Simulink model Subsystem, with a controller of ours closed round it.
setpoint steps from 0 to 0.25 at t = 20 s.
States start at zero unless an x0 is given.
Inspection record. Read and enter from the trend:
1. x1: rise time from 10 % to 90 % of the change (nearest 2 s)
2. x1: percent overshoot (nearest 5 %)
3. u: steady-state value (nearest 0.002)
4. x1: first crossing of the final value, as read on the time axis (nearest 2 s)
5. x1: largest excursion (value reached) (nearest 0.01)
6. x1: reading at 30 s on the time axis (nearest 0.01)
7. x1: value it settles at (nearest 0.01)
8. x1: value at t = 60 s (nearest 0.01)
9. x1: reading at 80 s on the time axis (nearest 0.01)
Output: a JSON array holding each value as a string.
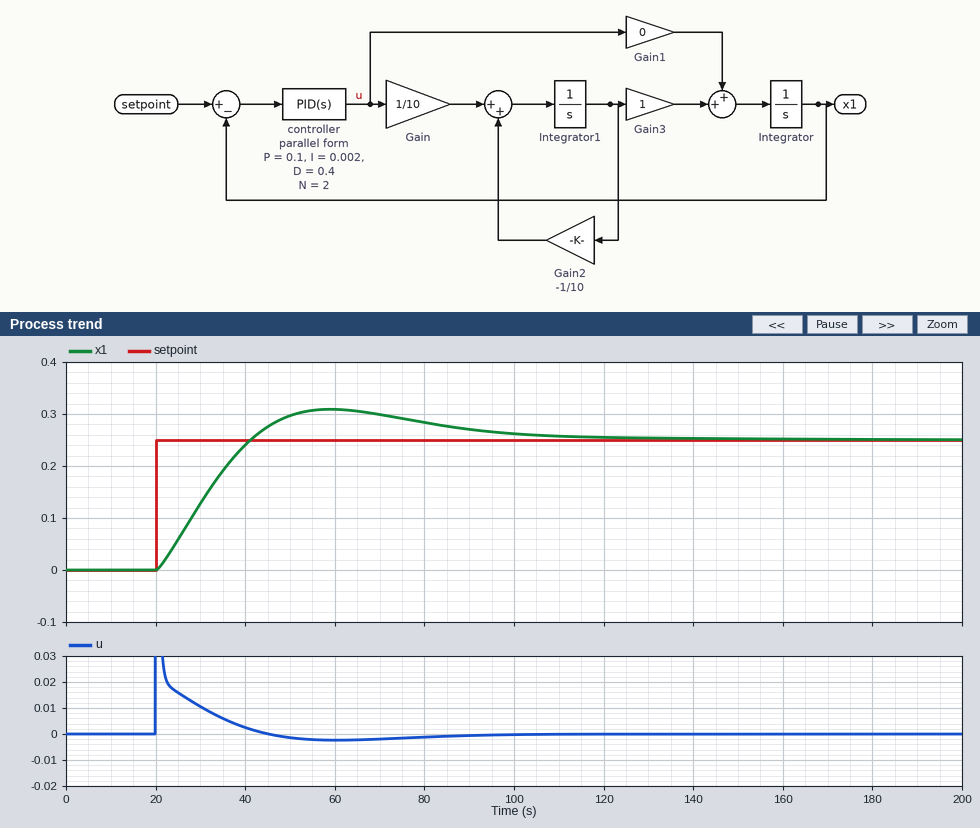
["16 s", "25 %", "0.000", "42 s", "0.31", "0.13", "0.25", "0.31", "0.28"]
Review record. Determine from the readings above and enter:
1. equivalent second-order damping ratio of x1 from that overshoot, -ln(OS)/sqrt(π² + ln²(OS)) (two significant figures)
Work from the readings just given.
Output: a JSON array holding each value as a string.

["0.40"]
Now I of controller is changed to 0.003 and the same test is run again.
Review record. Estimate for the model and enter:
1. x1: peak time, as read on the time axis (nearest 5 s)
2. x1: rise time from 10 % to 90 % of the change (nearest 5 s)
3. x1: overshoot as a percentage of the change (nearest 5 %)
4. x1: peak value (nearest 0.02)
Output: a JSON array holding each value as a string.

["60 s", "15 s", "30 %", "0.32"]
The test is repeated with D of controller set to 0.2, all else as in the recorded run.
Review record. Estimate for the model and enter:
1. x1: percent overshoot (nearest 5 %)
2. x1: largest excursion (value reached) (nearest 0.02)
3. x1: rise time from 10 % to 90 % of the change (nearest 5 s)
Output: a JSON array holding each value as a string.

["30 %", "0.32", "15 s"]
